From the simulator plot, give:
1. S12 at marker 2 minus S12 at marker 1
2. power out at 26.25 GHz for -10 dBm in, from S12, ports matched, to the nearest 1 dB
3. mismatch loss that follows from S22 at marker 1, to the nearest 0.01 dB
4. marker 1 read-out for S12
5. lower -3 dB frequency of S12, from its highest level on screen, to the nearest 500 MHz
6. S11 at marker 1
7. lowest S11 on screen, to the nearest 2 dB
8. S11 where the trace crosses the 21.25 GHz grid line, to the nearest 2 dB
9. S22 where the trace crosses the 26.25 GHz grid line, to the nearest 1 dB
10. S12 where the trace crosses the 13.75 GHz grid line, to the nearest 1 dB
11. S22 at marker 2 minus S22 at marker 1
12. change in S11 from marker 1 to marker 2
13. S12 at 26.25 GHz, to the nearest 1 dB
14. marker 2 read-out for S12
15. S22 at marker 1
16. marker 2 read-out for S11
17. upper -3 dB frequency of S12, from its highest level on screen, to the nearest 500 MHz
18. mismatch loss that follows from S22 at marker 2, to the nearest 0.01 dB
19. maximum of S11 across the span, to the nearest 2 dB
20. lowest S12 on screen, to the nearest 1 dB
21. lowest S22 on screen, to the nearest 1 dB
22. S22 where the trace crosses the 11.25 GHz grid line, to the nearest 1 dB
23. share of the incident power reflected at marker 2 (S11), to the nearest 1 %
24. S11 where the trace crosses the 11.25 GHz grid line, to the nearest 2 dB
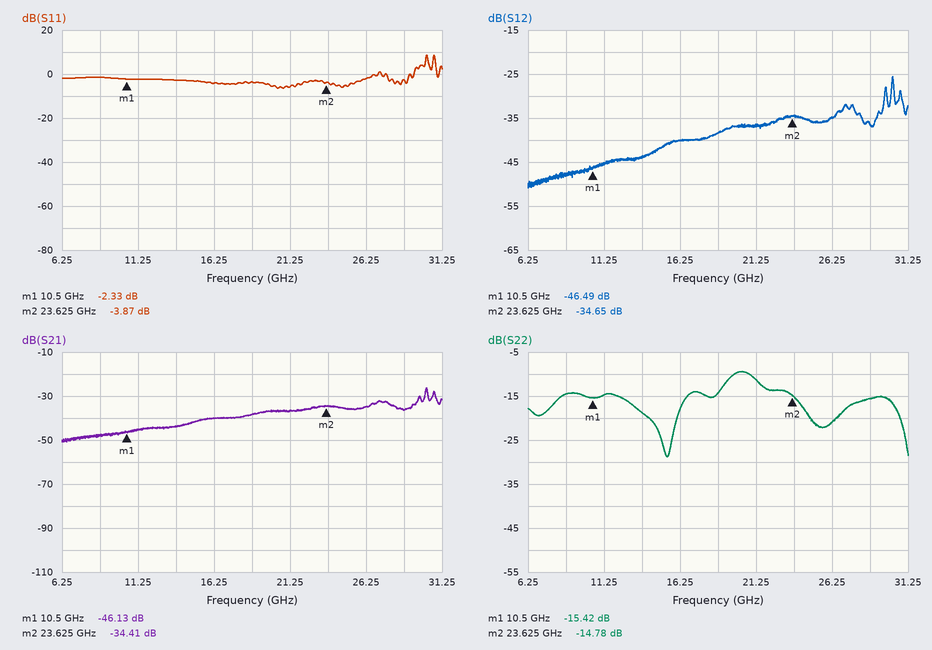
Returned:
11.84 dB
-45 dBm
0.13 dB
-46.49 dB
30.0 GHz
-2.33 dB
-6 dB
-6 dB
-21 dB
-44 dB
0.64 dB
-1.54 dB
-35 dB
-34.65 dB
-15.42 dB
-3.87 dB
30.5 GHz
0.15 dB
8 dB
-51 dB
-29 dB
-15 dB
41 %
-2 dB
